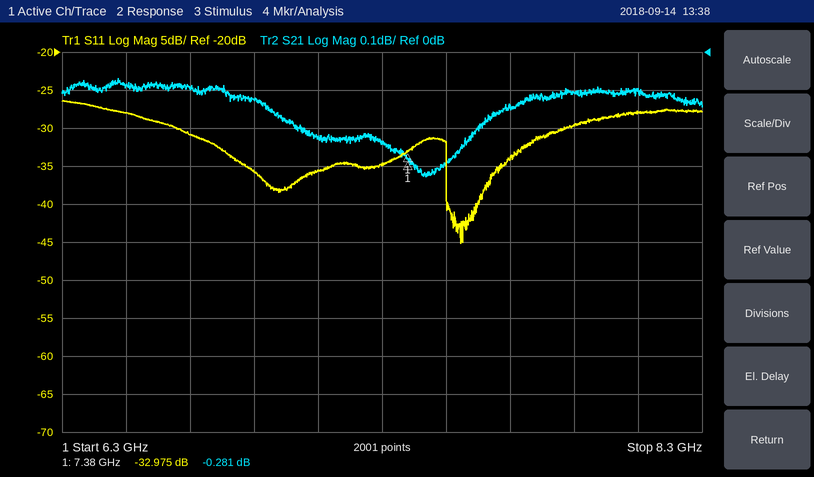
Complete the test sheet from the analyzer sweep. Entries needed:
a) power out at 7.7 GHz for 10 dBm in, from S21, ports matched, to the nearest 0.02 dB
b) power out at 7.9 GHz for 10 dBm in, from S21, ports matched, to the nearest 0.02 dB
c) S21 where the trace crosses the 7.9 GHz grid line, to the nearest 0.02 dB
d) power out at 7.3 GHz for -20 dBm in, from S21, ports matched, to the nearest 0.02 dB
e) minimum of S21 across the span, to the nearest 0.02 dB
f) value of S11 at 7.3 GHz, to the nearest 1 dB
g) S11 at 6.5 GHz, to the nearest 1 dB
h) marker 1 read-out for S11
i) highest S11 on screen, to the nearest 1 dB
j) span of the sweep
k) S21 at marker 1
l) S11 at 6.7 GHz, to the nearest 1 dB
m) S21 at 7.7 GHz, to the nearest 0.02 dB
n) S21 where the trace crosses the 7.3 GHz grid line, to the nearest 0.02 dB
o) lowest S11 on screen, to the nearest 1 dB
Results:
9.86 dBm
9.90 dBm
-0.10 dB
-20.24 dBm
-0.32 dB
-35 dB
-28 dB
-32.975 dB
-26 dB
2 GHz
-0.281 dB
-31 dB
-0.14 dB
-0.24 dB
-45 dB
